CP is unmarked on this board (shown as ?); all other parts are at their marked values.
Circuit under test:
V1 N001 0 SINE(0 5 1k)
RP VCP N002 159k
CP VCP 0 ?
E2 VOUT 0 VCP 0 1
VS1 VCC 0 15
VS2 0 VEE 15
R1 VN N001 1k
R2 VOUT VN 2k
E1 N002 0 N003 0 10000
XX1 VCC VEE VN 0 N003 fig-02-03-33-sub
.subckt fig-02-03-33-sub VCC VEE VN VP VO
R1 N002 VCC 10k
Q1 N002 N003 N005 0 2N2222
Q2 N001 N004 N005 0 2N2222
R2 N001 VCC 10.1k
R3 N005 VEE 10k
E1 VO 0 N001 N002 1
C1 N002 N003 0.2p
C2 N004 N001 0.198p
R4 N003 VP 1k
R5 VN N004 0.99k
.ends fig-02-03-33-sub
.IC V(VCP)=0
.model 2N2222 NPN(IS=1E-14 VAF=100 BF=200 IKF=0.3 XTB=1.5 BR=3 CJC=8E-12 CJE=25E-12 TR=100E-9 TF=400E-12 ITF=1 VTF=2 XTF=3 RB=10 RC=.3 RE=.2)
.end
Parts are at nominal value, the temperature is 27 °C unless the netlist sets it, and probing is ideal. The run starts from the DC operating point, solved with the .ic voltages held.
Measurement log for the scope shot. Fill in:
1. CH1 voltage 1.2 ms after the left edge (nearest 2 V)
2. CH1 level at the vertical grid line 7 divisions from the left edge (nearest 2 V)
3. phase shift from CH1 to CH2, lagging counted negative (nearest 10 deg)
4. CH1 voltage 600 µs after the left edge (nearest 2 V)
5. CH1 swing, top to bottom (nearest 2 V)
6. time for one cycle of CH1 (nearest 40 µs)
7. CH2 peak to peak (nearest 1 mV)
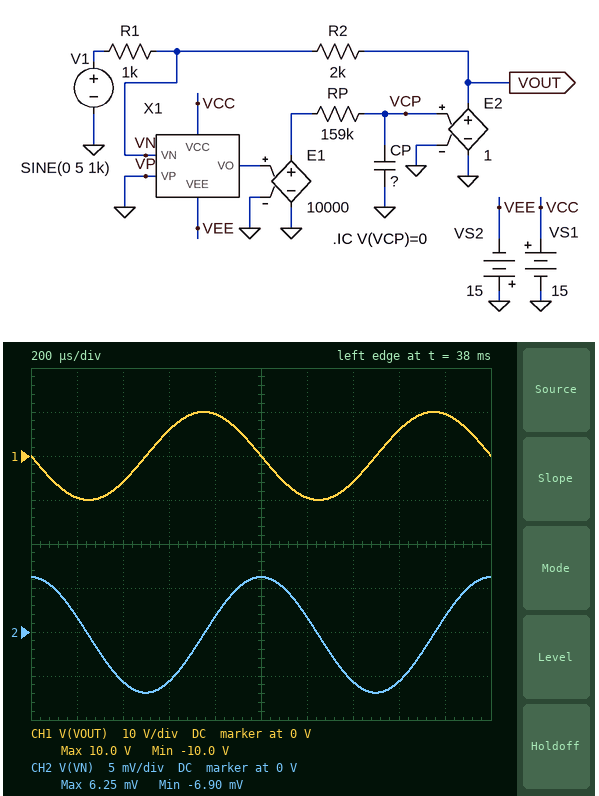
-10 V
-6 V
-90 deg
6 V
20 V
1.00 ms
13 mV
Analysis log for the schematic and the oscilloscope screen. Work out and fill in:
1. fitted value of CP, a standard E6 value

1.5 µF
